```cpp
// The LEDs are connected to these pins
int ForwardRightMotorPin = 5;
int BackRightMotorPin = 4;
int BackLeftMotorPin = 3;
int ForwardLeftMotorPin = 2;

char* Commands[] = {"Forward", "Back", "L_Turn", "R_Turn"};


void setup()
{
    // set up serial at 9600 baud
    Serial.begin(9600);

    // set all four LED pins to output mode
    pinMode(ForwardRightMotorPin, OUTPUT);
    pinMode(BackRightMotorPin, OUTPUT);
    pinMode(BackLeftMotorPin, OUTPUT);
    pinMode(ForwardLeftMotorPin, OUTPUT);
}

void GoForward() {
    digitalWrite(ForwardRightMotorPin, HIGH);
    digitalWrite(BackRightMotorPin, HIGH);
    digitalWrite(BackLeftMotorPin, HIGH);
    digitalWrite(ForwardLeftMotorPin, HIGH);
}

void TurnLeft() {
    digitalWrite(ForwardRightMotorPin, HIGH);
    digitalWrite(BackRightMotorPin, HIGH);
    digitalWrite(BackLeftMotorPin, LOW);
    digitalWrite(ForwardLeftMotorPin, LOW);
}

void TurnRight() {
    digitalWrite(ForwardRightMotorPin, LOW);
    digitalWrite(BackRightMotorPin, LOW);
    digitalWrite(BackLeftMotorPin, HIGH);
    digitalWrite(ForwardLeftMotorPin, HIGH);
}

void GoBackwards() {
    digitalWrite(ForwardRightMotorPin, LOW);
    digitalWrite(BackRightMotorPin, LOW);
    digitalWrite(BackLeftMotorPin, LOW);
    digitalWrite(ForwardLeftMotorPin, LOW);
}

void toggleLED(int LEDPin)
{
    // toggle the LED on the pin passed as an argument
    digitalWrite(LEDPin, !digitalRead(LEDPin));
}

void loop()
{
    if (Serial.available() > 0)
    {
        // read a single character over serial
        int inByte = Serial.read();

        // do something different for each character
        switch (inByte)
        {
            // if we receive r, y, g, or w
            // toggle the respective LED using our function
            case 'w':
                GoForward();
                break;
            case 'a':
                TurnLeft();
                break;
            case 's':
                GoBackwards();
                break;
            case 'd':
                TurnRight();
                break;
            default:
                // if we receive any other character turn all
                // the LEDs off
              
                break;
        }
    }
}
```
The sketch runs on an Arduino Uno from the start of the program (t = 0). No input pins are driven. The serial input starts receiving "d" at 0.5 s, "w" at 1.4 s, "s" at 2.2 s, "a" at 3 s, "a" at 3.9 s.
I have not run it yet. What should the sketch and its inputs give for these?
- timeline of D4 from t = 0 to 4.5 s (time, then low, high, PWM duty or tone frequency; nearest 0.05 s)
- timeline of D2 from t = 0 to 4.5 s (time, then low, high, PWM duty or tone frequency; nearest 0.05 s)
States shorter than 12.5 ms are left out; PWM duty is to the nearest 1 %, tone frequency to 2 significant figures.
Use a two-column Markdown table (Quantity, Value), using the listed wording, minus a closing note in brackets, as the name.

| Quantity | Value |
|---|---|
| timeline of D4 from t = 0 to 4.5 s | 0 s low; 1.4 s high; 2.2 s low; 3 s high |
| timeline of D2 from t = 0 to 4.5 s | 0 s low; 0.5 s high; 2.2 s low |
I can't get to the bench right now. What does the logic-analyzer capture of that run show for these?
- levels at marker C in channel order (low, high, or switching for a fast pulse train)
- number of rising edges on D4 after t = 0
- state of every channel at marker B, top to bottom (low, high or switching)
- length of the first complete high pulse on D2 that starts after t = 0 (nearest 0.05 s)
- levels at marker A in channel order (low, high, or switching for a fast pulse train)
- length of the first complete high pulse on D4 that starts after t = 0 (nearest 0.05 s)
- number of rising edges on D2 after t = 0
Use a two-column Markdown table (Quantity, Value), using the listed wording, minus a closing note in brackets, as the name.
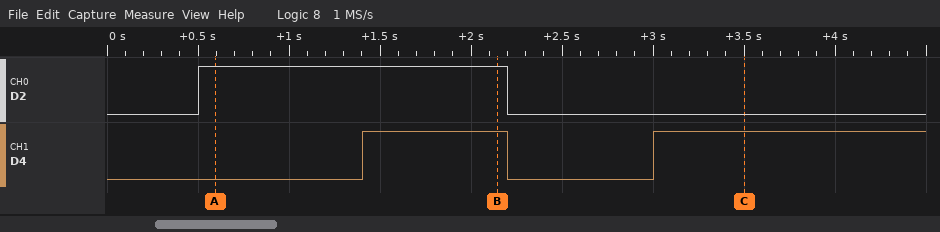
| Quantity | Value |
|---|---|
| levels at marker C in channel order | D2 low, D4 high |
| number of rising edges on D4 after t = 0 | 2 |
| state of every channel at marker B, top to bottom | D2 high, D4 high |
| length of the first complete high pulse on D2 that starts after t = 0 | 1.70 s |
| levels at marker A in channel order | D2 high, D4 low |
| length of the first complete high pulse on D4 that starts after t = 0 | 0.80 s |
| number of rising edges on D2 after t = 0 | 1 |
